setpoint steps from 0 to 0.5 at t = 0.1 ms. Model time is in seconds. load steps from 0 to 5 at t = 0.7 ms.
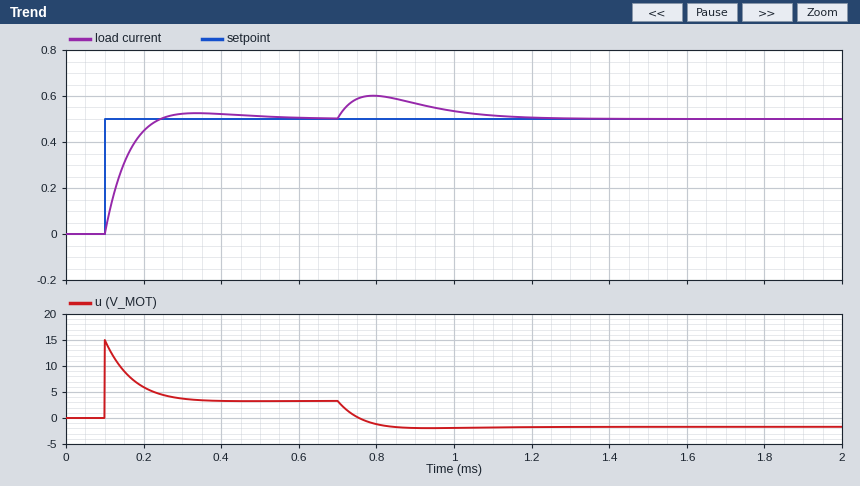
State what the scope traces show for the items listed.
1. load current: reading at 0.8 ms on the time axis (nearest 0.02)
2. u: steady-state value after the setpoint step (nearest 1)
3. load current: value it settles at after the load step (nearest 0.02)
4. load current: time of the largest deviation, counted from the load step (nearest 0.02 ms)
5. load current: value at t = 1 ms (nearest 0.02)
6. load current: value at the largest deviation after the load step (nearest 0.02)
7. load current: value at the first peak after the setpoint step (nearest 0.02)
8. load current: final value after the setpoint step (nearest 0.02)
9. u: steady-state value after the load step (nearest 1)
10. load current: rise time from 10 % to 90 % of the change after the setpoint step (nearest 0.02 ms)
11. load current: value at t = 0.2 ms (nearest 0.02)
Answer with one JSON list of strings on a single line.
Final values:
["0.60", "3", "0.50", "0.10 ms", "0.54", "0.60", "0.52", "0.50", "-2", "0.10 ms", "0.44"]
